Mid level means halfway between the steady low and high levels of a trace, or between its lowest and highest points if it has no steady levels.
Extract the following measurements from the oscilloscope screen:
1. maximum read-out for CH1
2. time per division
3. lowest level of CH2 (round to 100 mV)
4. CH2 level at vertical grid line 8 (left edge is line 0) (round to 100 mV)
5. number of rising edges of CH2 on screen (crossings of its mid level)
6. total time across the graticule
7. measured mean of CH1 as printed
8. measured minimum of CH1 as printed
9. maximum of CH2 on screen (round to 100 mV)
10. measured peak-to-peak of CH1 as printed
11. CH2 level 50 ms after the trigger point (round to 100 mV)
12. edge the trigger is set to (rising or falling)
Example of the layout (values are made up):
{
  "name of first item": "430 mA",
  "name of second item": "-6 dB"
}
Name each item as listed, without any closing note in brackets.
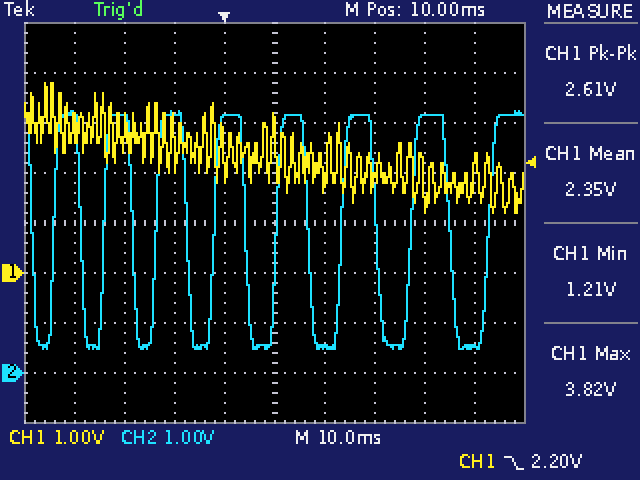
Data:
{
  "maximum read-out for CH1": "3.82 V",
  "time per division": "10 ms",
  "lowest level of CH2": "500 mV",
  "CH2 level at vertical grid line 8 (left edge is line 0)": "5.1 V",
  "number of rising edges of CH2 on screen": "8",
  "total time across the graticule": "100 ms",
  "measured mean of CH1 as printed": "2.35 V",
  "measured minimum of CH1 as printed": "1.21 V",
  "maximum of CH2 on screen": "5.2 V",
  "measured peak-to-peak of CH1 as printed": "2.61 V",
  "CH2 level 50 ms after the trigger point": "500 mV",
  "edge the trigger is set to": "falling"
}
